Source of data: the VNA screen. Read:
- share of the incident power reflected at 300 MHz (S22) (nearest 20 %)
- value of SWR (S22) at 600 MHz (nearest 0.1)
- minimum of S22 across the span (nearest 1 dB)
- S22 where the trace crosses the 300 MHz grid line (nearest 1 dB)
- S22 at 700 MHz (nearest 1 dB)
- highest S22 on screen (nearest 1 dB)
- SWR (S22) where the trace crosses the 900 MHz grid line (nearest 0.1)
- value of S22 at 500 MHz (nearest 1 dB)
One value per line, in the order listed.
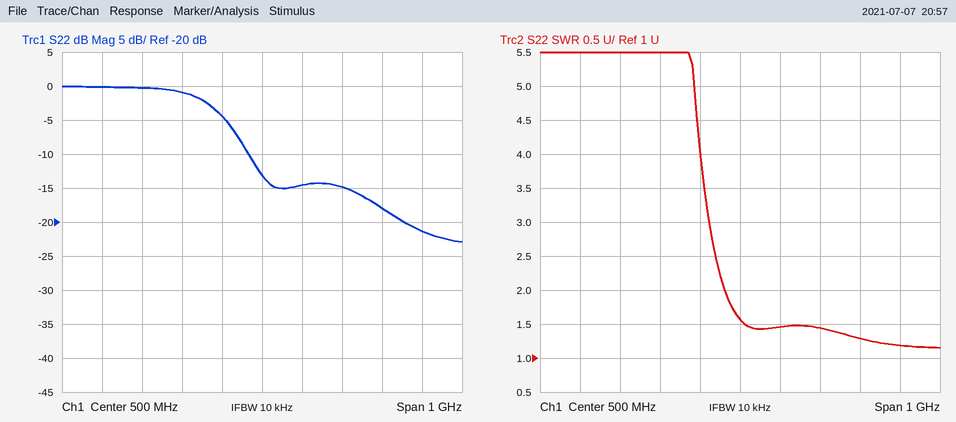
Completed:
80 %
1.5
-23 dB
-1 dB
-15 dB
0 dB
1.2
-13 dB
